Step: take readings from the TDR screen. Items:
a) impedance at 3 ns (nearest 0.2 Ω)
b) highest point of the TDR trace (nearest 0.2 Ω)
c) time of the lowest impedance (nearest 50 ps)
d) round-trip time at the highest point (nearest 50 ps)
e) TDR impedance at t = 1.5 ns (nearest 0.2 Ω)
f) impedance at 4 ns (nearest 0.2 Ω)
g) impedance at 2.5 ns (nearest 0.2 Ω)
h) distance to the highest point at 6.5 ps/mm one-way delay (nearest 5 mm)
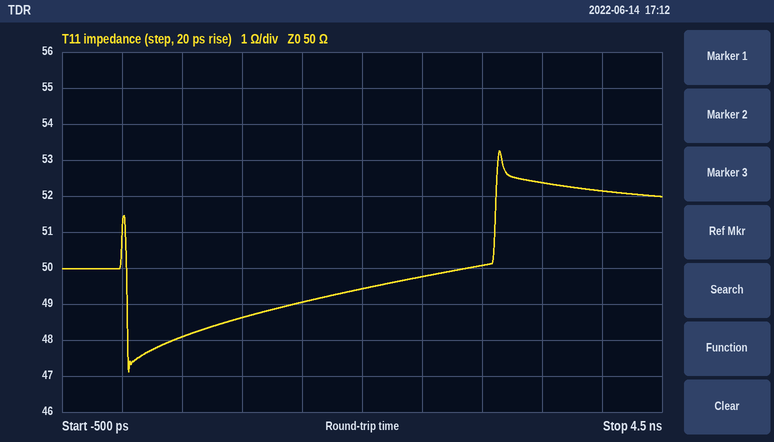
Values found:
50.0 Ω
53.2 Ω
50 ps
3.15 ns
49.0 Ω
52.2 Ω
49.8 Ω
240 mm
